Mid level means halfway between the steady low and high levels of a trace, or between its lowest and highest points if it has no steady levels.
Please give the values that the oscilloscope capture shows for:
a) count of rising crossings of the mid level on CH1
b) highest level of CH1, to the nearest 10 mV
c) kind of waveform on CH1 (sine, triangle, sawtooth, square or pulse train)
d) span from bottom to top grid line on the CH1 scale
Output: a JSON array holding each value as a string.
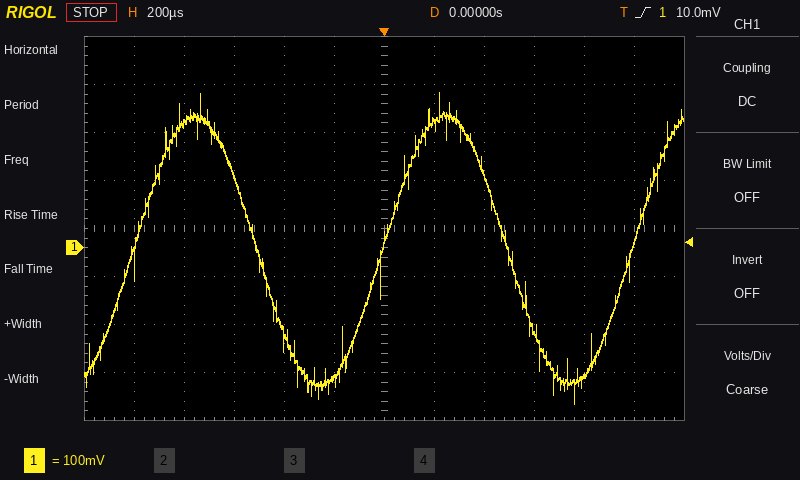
["3", "320 mV", "sine", "800 mV"]
